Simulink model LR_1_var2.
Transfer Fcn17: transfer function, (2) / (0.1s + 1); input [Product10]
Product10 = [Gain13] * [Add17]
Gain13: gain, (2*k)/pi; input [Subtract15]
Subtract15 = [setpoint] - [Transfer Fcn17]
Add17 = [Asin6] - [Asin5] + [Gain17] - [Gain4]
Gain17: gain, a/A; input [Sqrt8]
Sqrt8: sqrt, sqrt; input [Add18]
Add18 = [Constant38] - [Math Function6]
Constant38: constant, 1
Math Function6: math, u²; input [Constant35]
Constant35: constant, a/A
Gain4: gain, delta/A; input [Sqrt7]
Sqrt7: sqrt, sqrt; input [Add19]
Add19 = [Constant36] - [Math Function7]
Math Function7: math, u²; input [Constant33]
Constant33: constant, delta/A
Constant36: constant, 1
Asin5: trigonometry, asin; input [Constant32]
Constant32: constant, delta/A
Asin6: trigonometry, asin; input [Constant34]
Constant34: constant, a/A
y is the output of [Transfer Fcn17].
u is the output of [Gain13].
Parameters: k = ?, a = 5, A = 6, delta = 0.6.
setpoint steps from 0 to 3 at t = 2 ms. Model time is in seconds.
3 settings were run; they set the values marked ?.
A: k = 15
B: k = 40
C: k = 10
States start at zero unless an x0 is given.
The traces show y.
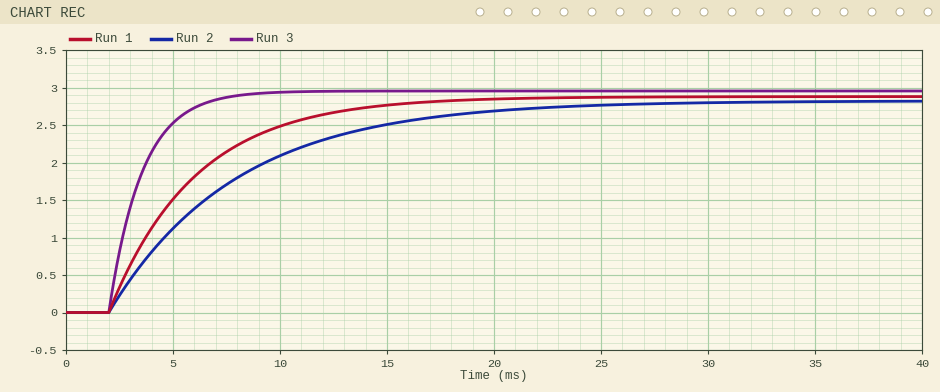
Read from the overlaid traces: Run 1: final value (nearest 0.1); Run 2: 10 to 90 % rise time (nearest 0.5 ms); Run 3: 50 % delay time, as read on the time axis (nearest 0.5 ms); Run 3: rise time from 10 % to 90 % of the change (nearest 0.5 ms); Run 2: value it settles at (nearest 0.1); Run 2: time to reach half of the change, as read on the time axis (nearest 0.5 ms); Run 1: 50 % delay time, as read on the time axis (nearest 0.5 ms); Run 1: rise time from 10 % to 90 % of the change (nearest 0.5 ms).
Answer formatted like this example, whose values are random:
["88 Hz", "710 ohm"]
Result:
["2.9", "13.0 ms", "3.0 ms", "3.5 ms", "2.8", "6.0 ms", "5.0 ms", "9.0 ms"]
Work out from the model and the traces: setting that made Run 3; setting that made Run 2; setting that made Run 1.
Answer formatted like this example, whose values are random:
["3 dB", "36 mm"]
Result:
["B", "C", "A"]
